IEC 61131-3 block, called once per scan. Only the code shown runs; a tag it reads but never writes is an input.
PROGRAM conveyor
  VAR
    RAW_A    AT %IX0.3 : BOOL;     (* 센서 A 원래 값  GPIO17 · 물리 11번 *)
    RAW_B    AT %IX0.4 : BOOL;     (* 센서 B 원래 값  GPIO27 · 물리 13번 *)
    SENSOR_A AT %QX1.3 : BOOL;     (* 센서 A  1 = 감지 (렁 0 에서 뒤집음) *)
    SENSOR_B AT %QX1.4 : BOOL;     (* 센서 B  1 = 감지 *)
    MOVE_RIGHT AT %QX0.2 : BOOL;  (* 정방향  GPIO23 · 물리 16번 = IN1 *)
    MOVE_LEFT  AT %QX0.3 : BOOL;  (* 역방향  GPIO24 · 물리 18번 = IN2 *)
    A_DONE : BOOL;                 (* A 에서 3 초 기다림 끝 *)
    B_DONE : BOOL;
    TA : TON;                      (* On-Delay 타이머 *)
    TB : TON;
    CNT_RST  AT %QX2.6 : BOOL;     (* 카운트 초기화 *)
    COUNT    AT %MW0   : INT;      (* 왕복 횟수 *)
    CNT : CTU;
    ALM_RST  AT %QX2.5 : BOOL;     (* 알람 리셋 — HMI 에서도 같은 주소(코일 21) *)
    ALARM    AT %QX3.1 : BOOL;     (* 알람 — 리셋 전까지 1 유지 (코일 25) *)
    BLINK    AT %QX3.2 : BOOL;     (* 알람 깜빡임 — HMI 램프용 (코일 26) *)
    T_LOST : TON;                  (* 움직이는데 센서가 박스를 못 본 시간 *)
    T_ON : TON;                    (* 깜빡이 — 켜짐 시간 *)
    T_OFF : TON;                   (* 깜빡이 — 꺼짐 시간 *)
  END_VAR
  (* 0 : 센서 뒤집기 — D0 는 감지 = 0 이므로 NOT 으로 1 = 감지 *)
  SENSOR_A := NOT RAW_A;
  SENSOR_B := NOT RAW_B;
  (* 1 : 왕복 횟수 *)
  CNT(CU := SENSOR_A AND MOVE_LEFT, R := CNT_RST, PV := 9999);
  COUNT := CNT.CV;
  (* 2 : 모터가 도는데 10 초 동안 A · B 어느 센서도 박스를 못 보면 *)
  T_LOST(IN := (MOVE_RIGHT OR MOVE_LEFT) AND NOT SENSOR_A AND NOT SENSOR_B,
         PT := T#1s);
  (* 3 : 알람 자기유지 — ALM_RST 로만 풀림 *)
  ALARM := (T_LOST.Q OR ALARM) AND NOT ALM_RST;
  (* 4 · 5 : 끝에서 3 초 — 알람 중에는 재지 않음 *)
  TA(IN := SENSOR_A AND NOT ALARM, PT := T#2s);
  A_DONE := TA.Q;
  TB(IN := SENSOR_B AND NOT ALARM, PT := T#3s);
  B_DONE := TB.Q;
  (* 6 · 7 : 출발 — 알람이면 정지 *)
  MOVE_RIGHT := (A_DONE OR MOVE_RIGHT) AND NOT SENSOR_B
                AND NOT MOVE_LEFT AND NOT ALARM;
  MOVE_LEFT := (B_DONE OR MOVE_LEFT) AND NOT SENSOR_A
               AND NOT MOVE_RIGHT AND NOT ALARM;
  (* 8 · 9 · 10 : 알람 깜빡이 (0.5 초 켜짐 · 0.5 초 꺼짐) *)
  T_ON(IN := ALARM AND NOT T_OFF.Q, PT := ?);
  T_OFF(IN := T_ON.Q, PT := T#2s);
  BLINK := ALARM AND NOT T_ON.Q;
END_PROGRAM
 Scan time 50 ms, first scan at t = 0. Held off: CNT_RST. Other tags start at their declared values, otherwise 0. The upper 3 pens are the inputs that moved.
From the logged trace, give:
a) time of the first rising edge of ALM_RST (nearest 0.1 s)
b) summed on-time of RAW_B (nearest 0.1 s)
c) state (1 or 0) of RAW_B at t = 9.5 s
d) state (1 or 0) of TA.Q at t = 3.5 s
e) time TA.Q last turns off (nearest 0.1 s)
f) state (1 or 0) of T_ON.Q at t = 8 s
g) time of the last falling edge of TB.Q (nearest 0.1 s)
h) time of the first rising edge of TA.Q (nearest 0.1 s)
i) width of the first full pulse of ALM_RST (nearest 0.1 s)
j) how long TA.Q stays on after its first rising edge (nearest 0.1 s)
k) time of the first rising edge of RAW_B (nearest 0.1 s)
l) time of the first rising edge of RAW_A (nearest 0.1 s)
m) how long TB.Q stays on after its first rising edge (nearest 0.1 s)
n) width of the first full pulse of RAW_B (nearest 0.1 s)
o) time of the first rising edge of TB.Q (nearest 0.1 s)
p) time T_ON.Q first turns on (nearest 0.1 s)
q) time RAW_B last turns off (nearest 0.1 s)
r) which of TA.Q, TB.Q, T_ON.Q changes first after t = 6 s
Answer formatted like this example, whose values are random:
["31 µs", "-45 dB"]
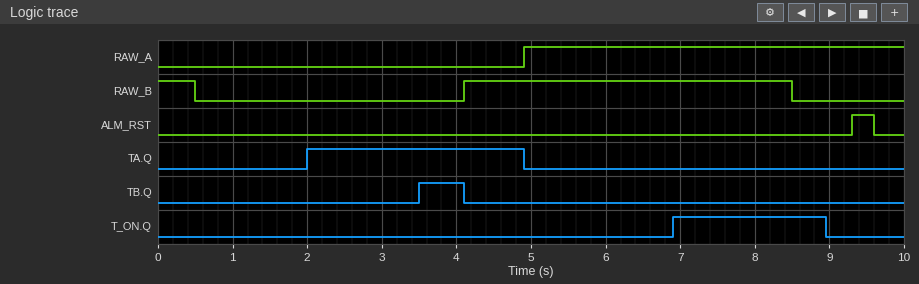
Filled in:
["9.3 s", "4.9 s", "0", "1", "4.9 s", "1", "4.1 s", "2.0 s", "0.3 s", "2.9 s", "4.1 s", "4.9 s", "0.6 s", "4.4 s", "3.5 s", "6.9 s", "8.5 s", "T_ON.Q"]
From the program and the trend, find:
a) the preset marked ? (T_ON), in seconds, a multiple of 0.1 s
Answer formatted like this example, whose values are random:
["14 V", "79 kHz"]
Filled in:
["1.0 s"]
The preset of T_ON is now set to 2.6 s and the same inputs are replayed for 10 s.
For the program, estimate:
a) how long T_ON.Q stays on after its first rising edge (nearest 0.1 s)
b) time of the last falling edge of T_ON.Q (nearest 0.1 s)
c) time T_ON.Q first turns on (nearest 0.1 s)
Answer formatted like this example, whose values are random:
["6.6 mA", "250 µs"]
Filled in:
["0.8 s", "9.3 s", "8.5 s"]
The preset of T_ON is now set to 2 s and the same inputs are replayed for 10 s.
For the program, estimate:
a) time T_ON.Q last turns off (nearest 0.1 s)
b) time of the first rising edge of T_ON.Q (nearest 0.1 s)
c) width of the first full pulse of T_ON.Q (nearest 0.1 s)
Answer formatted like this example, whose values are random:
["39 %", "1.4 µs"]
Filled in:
["9.3 s", "7.9 s", "1.4 s"]
